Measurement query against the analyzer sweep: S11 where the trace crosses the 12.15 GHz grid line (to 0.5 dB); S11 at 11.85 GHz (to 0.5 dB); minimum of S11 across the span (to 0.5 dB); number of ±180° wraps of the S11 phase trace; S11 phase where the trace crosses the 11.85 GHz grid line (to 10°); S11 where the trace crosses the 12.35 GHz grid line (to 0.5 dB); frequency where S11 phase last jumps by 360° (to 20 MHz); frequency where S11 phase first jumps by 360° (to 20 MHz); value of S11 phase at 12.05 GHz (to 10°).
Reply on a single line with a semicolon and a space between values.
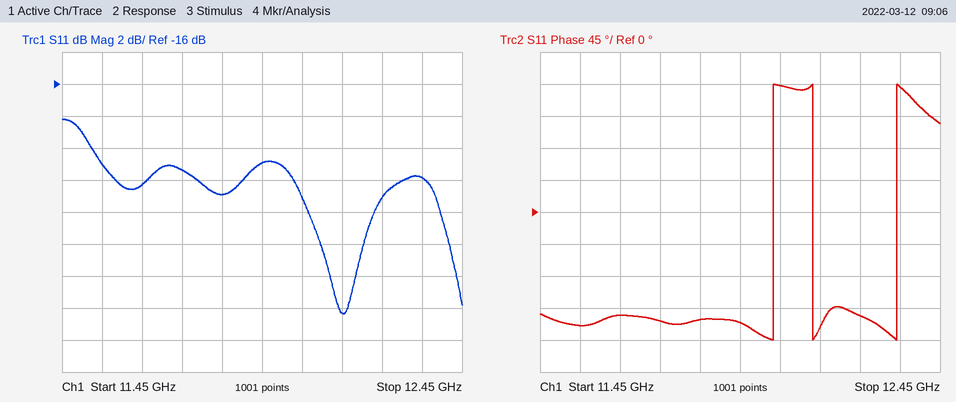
-30.5 dB; -23.0 dB; -30.5 dB; 3; -150°; -22.0 dB; 12.34 GHz; 12.04 GHz; 180°
